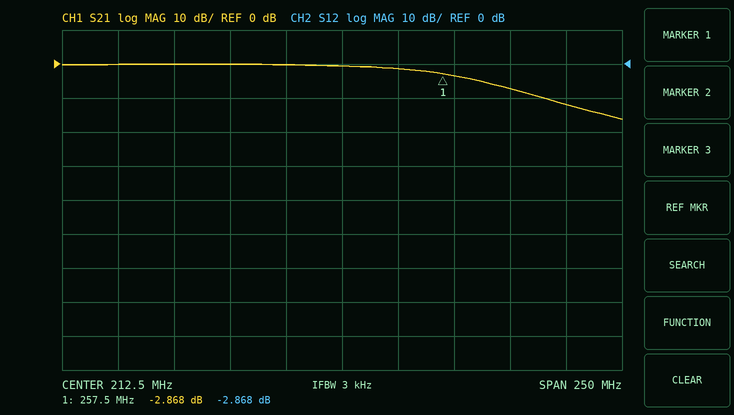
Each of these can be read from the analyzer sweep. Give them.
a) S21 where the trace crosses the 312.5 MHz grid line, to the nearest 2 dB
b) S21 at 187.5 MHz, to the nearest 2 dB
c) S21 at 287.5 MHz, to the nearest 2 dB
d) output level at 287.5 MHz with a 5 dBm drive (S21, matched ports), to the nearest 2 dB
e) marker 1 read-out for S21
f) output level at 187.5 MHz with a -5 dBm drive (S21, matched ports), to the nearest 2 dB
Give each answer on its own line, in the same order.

-12 dB
0 dB
-8 dB
-2 dBm
-2.868 dB
-6 dBm
